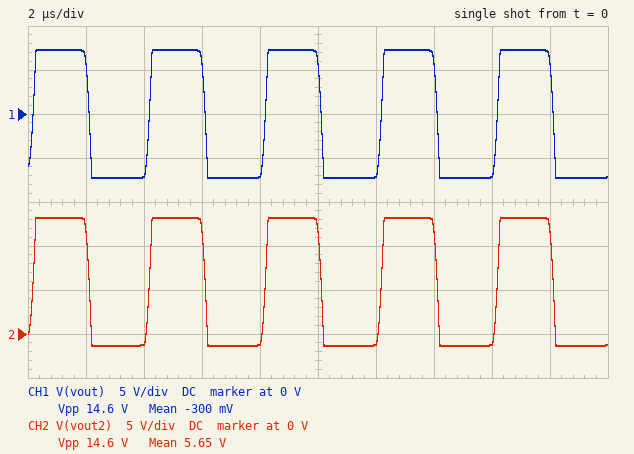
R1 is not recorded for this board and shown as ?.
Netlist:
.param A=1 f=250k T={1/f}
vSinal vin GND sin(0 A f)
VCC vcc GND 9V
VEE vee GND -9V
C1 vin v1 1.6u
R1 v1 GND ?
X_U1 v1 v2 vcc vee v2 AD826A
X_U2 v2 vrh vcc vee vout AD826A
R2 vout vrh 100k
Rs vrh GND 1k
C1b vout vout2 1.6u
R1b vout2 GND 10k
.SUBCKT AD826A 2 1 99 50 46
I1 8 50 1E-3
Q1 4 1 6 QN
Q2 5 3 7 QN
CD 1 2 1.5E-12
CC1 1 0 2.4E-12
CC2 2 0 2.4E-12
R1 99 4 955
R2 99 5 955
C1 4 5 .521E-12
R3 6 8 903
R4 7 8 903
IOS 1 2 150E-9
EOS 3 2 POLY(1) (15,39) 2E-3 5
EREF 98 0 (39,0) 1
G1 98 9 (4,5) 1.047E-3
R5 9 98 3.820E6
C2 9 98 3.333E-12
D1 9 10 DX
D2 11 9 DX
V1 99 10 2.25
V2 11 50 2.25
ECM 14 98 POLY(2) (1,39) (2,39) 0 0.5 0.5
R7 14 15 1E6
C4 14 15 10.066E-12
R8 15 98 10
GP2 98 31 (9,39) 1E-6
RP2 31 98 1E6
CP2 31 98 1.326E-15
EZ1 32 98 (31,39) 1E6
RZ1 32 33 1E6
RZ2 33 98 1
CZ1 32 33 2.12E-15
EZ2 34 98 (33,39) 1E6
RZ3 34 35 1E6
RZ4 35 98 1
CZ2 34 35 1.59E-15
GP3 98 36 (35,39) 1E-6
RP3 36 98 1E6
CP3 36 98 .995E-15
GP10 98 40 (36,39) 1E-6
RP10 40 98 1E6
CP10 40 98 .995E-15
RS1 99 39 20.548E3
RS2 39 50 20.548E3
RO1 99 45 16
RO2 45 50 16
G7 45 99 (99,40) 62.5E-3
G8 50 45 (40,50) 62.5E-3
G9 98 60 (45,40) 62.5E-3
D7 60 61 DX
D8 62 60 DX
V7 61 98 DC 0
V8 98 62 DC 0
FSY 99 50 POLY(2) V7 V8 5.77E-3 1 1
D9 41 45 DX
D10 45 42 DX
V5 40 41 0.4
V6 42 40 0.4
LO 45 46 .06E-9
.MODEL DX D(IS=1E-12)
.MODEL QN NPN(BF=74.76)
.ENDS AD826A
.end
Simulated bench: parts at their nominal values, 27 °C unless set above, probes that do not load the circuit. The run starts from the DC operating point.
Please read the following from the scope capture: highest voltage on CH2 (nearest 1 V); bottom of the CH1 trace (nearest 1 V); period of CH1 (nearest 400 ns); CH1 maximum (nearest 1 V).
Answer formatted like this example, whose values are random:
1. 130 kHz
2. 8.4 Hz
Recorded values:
1. 13 V
2. -7 V
3. 4.0 µs
4. 7 V
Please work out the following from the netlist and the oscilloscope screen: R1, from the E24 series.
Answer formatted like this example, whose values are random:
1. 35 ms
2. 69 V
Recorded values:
1. 11 kΩ
